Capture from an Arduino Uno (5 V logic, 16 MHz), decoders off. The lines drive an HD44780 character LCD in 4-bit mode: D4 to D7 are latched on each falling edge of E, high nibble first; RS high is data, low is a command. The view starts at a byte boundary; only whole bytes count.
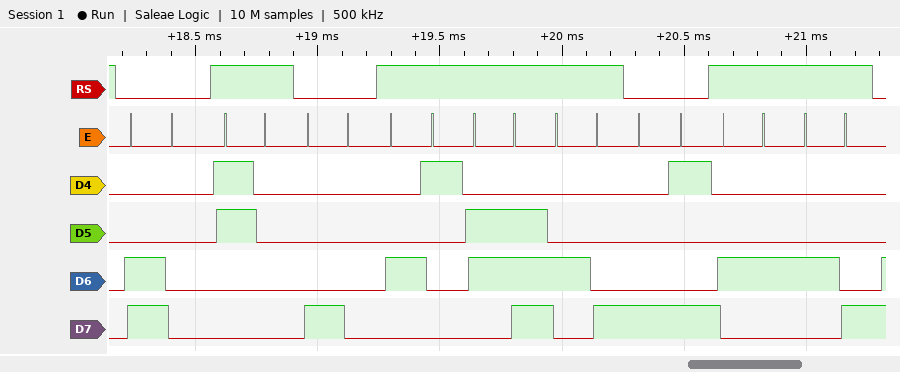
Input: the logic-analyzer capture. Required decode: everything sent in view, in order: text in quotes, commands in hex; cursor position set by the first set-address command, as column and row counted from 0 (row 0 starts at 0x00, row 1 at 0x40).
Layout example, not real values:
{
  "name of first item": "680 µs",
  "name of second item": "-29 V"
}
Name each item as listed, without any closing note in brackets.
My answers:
{
  "everything sent in view, in order: text in quotes, commands in hex": "0xC0 \"0\" 0x80 \"AnH\" 0x89 \"DH\"",
  "cursor position set by the first set-address command, as column and row counted from 0": "column 0, row 1"
}
